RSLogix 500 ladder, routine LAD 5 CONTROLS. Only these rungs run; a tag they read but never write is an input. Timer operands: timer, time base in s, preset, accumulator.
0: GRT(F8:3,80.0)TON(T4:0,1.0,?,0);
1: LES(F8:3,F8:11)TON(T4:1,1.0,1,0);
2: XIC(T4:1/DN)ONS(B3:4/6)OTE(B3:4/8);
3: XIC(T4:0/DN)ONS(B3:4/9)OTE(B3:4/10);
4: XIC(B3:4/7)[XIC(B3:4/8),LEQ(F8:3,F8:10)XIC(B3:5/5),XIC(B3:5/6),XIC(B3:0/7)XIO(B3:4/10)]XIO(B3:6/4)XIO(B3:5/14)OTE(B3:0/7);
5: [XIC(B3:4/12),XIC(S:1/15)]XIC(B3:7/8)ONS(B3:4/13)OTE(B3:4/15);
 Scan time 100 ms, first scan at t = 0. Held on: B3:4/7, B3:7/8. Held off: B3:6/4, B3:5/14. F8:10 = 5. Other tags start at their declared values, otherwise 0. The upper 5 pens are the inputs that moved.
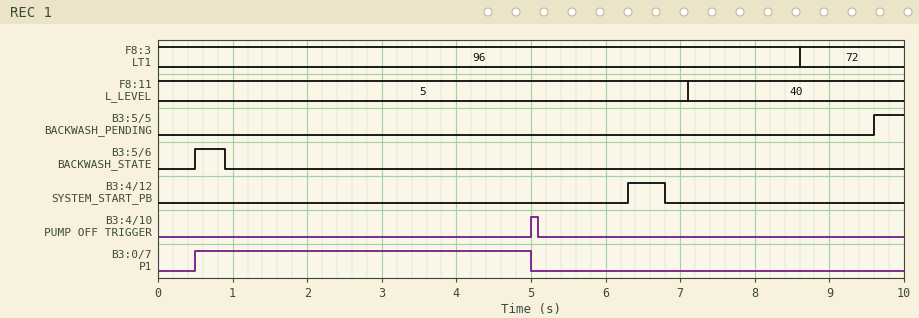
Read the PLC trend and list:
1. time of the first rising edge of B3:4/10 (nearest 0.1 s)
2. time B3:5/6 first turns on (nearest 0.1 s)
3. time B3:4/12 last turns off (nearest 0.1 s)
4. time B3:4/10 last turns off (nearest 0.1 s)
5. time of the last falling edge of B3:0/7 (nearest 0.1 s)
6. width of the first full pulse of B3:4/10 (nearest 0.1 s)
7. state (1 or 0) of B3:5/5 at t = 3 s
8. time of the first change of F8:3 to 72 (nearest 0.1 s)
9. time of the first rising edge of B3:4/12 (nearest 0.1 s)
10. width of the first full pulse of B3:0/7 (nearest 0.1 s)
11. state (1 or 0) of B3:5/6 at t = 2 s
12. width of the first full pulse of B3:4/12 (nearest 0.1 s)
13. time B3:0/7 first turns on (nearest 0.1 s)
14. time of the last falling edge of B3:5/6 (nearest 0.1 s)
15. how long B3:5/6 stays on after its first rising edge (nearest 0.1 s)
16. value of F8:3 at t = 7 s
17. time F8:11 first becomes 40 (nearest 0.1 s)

5.0 s
0.5 s
6.8 s
5.1 s
5.0 s
0.1 s
0
8.6 s
6.3 s
4.5 s
0
0.5 s
0.5 s
0.9 s
0.4 s
96
7.1 s
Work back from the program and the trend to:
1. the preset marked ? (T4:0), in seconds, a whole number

5 s
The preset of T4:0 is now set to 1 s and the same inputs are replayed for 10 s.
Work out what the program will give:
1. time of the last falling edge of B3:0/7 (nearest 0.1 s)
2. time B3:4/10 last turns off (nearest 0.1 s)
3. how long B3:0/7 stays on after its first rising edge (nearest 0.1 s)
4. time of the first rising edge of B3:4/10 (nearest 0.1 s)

1.0 s
1.1 s
0.5 s
1.0 s
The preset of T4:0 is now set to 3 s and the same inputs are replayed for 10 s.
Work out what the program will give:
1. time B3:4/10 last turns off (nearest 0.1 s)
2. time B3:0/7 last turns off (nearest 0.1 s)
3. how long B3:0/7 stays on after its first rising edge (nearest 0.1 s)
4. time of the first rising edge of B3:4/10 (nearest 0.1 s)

3.1 s
3.0 s
2.5 s
3.0 s
